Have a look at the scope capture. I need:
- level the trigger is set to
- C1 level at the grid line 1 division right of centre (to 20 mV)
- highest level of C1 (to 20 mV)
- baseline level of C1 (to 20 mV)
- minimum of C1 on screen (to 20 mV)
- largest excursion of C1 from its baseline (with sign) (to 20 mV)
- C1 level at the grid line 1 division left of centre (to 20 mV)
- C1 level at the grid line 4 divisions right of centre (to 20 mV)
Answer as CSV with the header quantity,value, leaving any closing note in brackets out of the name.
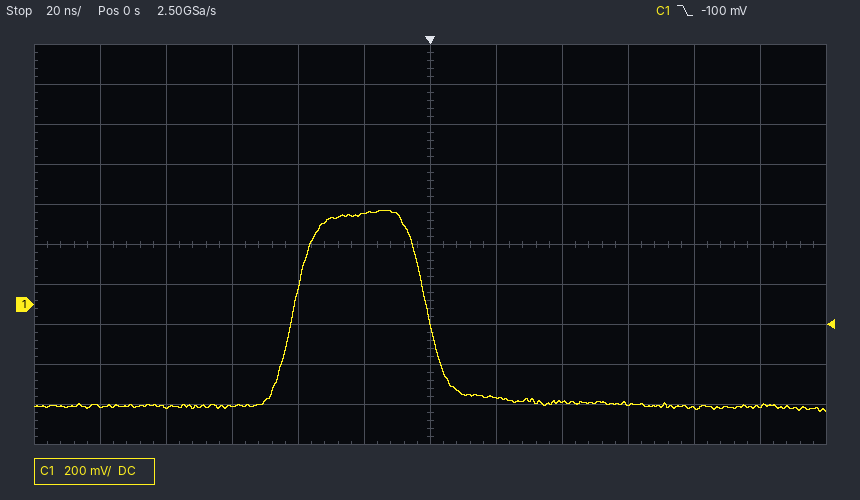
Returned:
quantity,value
level the trigger is set to,-100 mV
C1 level at the grid line 1 division right of centre,-460 mV
highest level of C1,480 mV
baseline level of C1,-500 mV
minimum of C1 on screen,-540 mV
largest excursion of C1 from its baseline (with sign),+980 mV
C1 level at the grid line 1 division left of centre,460 mV
C1 level at the grid line 4 divisions right of centre,-520 mV
